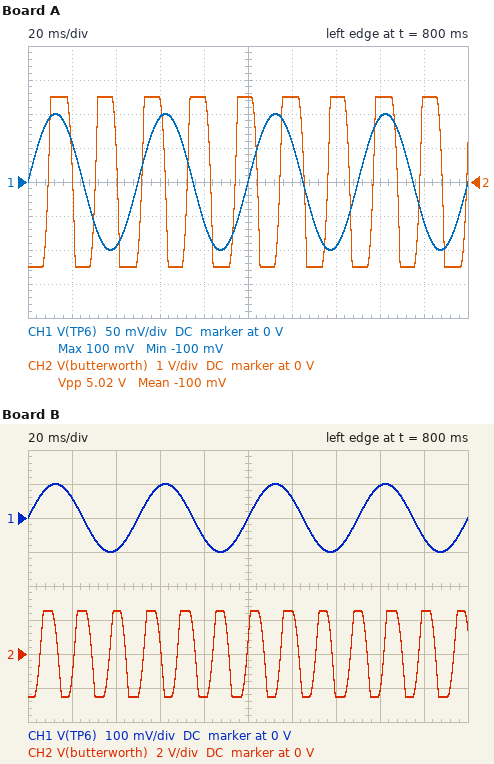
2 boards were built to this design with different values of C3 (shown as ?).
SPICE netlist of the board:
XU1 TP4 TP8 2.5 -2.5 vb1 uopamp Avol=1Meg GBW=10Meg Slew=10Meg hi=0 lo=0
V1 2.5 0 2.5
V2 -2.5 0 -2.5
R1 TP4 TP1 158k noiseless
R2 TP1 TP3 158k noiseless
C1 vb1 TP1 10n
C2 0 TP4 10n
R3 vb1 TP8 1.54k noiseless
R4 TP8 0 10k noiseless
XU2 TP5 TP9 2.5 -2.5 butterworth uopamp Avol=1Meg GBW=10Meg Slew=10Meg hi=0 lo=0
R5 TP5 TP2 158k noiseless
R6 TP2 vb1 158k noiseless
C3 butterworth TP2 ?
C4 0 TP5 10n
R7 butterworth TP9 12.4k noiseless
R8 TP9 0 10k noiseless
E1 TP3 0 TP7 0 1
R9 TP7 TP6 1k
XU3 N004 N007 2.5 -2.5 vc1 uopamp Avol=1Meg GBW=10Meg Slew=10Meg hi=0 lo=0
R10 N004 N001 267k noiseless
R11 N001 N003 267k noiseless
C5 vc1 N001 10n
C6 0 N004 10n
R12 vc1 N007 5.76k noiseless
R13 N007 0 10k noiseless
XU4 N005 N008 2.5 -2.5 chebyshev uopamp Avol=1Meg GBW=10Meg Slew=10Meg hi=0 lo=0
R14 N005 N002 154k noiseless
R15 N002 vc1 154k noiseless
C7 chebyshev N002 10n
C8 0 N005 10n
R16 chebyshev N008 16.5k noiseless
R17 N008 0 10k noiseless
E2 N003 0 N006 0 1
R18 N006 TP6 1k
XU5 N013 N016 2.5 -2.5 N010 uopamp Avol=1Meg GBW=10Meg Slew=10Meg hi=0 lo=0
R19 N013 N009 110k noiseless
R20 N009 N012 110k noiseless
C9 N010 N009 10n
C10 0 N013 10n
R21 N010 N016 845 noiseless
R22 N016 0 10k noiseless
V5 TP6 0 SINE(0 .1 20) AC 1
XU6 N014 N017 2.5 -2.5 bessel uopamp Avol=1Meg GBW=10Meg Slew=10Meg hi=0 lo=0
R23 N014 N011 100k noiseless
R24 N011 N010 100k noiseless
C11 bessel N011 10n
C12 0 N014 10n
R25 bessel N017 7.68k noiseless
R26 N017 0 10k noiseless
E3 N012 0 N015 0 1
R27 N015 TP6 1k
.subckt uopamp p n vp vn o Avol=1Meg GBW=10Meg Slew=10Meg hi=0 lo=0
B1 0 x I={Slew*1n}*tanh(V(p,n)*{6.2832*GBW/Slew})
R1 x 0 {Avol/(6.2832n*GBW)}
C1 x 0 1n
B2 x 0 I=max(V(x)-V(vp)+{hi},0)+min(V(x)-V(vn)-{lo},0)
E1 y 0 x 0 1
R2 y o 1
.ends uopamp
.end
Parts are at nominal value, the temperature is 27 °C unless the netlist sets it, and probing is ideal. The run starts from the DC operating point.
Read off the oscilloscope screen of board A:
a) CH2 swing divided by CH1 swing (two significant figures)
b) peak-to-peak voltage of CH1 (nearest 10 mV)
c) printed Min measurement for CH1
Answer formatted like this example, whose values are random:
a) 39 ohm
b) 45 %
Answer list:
a) 25
b) 200 mV
c) -100 mV
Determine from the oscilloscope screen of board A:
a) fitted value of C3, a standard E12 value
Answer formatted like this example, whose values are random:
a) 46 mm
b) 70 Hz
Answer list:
a) 33 nF
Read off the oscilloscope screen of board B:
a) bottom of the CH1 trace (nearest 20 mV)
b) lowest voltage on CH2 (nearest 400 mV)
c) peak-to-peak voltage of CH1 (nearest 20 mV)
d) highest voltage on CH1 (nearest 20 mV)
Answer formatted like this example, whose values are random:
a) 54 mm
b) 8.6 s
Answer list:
a) -100 mV
b) -2.4 V
c) 200 mV
d) 100 mV
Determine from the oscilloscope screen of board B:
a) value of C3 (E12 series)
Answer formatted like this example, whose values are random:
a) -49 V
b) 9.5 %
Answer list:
a) 22 nF
